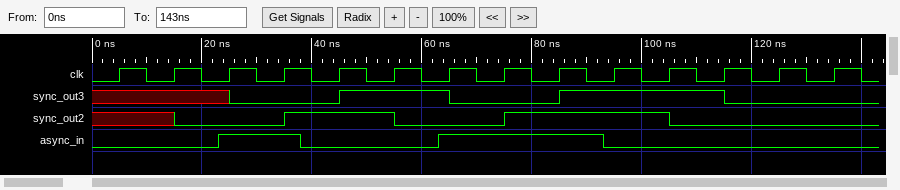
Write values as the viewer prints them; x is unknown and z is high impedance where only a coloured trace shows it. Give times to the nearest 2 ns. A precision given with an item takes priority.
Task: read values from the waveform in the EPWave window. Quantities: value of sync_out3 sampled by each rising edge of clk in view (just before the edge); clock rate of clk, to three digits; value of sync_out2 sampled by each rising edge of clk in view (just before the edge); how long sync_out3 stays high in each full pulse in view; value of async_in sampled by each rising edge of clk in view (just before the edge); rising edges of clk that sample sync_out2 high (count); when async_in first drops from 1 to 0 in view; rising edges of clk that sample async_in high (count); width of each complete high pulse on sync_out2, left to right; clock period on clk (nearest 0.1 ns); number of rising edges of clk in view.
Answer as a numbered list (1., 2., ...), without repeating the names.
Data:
1. x x x 0 0 1 1 0 0 1 1 1 0 0
2. 100 MHz
3. x x 0 0 1 1 0 0 1 1 1 0 0 0
4. 20 ns, 30 ns
5. 0 0 1 1 0 0 1 1 1 0 0 0 0 0
6. 5
7. 38 ns
8. 5
9. 20 ns, 30 ns
10. 10 ns
11. 14
